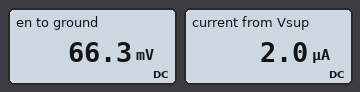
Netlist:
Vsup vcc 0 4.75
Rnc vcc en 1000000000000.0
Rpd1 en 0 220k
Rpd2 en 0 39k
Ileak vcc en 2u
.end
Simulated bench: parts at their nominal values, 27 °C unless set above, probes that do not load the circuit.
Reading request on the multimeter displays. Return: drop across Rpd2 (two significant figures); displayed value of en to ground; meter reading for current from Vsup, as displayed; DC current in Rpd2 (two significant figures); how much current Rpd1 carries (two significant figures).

66 mV
66.3 mV
2.0 µA
1.7 µA
300 nA
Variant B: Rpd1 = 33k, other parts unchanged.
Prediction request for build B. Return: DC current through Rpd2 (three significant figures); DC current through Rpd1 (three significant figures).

917 nA
1.08 µA
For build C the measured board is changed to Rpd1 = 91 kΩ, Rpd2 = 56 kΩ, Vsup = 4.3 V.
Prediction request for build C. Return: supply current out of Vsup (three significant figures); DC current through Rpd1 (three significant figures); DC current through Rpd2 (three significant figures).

2.00 µA
762 nA
1.24 µA
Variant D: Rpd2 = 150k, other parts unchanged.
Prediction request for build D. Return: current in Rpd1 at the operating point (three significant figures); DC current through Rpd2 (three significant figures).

811 nA
1.19 µA
